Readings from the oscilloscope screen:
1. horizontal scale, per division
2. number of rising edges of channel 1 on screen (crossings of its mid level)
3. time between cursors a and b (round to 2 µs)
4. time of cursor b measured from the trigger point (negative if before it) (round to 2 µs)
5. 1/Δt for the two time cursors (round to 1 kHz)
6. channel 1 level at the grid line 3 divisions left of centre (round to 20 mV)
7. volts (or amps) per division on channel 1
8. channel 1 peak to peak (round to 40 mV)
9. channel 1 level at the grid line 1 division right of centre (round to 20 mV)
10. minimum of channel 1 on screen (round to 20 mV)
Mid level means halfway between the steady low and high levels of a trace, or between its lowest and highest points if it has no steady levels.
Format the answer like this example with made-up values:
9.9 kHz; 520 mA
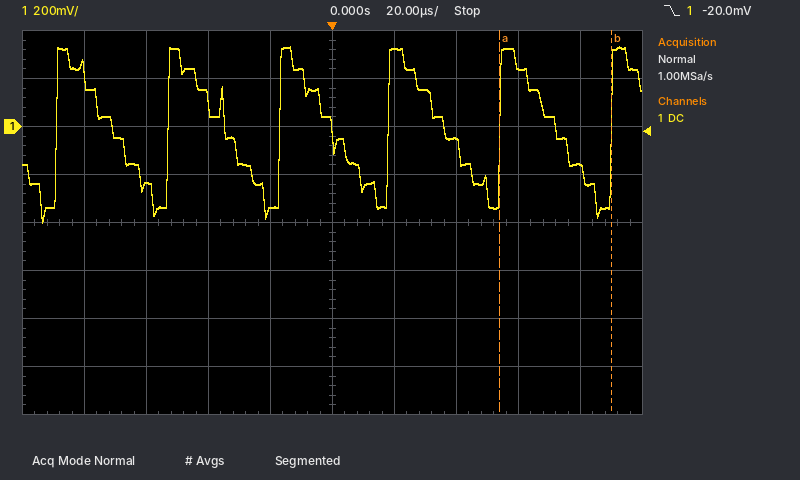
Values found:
20 µs; 6; 36 µs; +90 µs; 28 kHz; -240 mV; 200 mV; 720 mV; 320 mV; -400 mV
